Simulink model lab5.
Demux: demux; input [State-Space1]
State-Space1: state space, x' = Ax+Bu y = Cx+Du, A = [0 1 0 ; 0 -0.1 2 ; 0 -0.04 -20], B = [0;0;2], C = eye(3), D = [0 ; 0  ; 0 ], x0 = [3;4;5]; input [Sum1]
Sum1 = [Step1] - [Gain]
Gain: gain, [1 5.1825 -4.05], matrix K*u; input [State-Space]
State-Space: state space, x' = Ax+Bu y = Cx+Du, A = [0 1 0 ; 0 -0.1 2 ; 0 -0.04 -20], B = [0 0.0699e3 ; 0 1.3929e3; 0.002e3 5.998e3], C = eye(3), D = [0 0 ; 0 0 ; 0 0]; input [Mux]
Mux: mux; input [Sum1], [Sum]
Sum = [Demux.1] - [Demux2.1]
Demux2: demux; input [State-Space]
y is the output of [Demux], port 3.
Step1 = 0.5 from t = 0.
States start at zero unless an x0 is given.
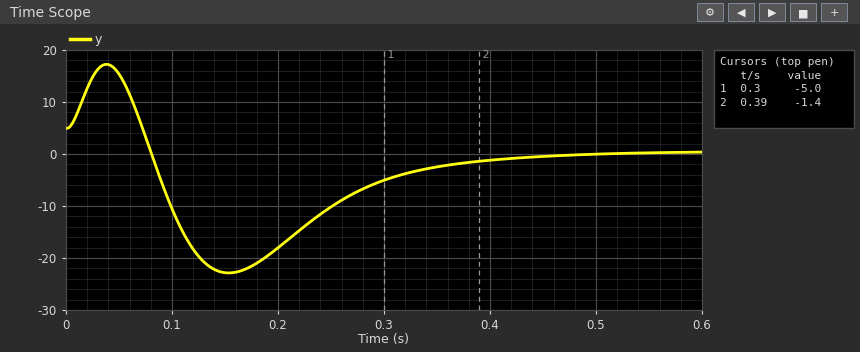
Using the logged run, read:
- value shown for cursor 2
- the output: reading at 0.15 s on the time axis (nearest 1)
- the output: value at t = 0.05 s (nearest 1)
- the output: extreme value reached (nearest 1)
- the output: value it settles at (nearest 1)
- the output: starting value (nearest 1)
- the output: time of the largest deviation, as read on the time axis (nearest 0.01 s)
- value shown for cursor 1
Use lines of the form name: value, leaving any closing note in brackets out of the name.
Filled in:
value shown for cursor 2: -1.4
the output: reading at 0.15 s on the time axis: -23
the output: value at t = 0.05 s: 15
the output: extreme value reached: -23
the output: value it settles at: 0
the output: starting value: 5
the output: time of the largest deviation, as read on the time axis: 0.15 s
value shown for cursor 1: -5.0
